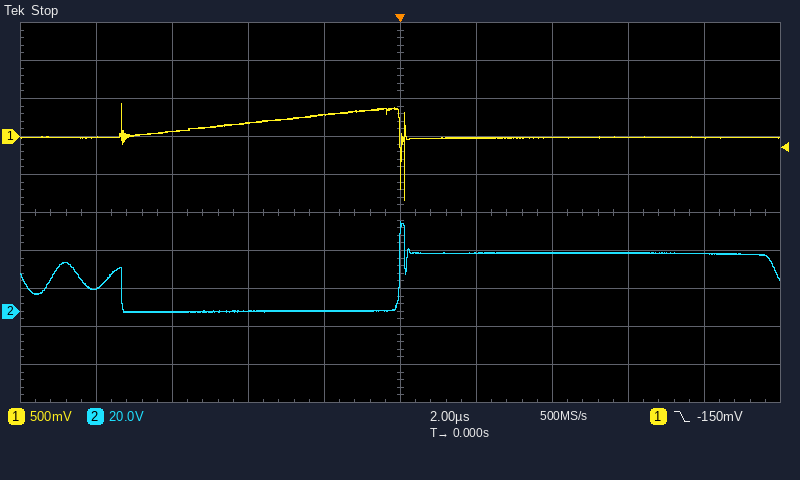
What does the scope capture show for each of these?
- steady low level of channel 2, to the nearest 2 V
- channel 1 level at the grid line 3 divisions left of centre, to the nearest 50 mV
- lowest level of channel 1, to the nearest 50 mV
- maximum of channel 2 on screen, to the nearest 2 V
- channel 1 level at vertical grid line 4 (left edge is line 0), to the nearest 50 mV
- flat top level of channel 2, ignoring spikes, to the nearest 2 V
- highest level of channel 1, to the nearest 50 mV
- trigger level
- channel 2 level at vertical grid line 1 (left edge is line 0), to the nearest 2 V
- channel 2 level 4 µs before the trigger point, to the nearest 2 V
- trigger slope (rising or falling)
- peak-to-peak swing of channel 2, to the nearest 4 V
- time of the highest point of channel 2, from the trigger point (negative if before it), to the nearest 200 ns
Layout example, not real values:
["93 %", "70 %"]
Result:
["0 V", "50 mV", "-850 mV", "48 V", "300 mV", "30 V", "450 mV", "-150 mV", "12 V", "0 V", "falling", "48 V", "0.0 µs"]
